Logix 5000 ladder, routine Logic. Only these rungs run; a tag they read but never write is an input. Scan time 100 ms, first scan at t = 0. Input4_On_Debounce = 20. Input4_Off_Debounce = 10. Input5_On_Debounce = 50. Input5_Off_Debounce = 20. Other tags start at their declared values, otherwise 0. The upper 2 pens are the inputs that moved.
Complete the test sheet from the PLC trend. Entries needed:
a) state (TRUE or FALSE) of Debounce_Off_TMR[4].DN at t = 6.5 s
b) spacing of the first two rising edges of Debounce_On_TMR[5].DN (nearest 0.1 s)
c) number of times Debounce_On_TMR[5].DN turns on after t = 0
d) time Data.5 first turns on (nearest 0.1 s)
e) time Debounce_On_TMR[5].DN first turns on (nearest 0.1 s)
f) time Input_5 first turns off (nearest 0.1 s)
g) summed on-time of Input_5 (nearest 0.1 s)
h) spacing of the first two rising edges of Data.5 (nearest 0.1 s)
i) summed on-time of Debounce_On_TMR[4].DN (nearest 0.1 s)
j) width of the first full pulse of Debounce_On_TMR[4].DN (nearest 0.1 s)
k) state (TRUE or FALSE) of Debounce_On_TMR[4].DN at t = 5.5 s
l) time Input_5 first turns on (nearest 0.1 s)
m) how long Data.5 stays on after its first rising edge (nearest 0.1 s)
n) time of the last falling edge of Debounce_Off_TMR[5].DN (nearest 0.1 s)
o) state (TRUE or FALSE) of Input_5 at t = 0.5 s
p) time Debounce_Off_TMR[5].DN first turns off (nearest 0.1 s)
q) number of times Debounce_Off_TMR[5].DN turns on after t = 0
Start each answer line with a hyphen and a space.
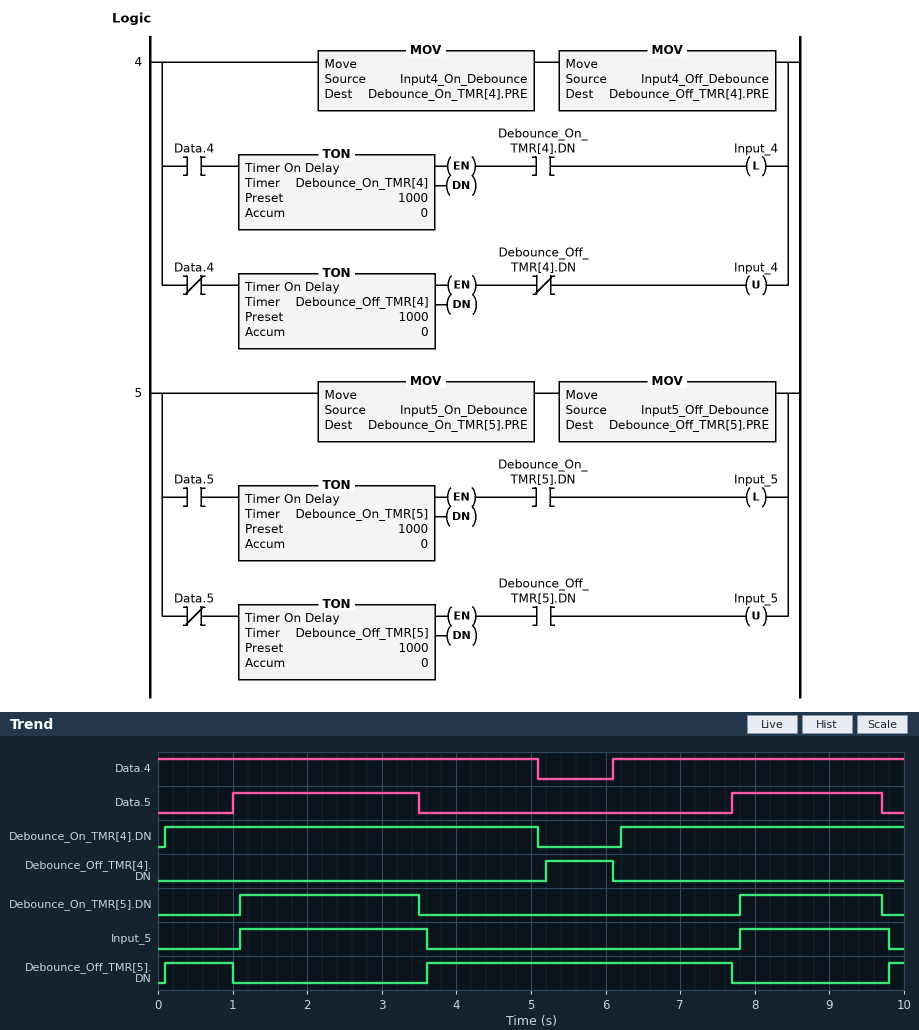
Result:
- FALSE
- 6.7 s
- 2
- 1.0 s
- 1.1 s
- 3.6 s
- 4.5 s
- 6.7 s
- 8.8 s
- 5.0 s
- FALSE
- 1.1 s
- 2.5 s
- 7.7 s
- FALSE
- 1.0 s
- 3
